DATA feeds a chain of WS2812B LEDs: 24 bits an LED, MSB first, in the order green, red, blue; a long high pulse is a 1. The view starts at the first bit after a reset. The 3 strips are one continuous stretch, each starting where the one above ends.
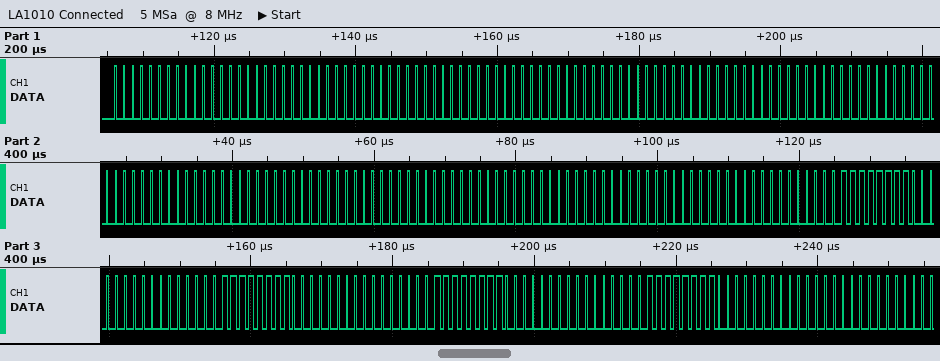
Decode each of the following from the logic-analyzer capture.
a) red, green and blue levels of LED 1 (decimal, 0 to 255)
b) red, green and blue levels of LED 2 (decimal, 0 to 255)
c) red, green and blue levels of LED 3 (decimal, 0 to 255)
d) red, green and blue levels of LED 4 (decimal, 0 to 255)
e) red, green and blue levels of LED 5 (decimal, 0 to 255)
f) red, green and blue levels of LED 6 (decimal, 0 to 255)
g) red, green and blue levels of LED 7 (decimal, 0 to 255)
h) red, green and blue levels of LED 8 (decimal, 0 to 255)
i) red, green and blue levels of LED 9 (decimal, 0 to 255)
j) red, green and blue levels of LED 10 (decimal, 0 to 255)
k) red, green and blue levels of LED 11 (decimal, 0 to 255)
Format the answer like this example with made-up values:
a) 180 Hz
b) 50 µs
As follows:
a) 0, 0, 0
b) 0, 0, 0
c) 0, 0, 0
d) 0, 0, 0
e) 0, 0, 0
f) 0, 0, 0
g) 0, 0, 0
h) 255, 0, 0
i) 255, 0, 0
j) 255, 0, 0
k) 255, 0, 0
